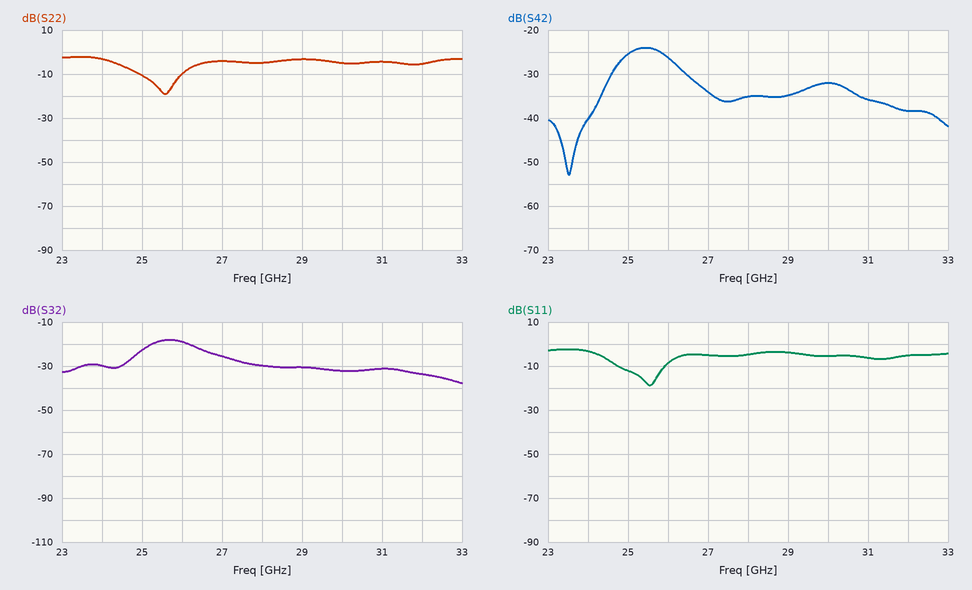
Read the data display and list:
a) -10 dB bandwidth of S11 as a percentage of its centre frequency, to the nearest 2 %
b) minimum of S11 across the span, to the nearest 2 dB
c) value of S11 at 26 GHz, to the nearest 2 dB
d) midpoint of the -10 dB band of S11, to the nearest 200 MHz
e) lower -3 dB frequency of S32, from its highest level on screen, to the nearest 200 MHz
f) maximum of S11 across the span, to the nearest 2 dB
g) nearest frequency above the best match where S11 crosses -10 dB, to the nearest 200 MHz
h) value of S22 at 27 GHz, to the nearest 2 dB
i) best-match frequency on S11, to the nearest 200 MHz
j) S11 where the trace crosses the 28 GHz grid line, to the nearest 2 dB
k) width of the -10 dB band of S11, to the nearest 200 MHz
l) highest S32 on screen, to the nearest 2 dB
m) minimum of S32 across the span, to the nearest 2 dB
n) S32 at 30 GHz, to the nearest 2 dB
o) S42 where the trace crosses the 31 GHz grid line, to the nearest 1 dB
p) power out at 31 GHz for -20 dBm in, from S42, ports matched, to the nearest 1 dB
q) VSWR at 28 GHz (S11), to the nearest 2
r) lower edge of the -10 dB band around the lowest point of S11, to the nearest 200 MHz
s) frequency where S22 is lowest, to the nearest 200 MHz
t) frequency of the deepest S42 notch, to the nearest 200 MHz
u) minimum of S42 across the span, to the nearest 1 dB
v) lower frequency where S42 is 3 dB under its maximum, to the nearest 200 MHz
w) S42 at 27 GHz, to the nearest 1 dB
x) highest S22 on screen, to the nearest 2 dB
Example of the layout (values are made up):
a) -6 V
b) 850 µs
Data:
a) 4 %
b) -18 dB
c) -8 dB
d) 25.4 GHz
e) 25.2 GHz
f) -2 dB
g) 26.0 GHz
h) -4 dB
i) 25.6 GHz
j) -4 dB
k) 1.2 GHz
l) -18 dB
m) -38 dB
n) -32 dB
o) -36 dB
p) -56 dBm
q) 4
r) 24.8 GHz
s) 25.6 GHz
t) 23.6 GHz
u) -53 dB
v) 24.8 GHz
w) -34 dB
x) -2 dB
